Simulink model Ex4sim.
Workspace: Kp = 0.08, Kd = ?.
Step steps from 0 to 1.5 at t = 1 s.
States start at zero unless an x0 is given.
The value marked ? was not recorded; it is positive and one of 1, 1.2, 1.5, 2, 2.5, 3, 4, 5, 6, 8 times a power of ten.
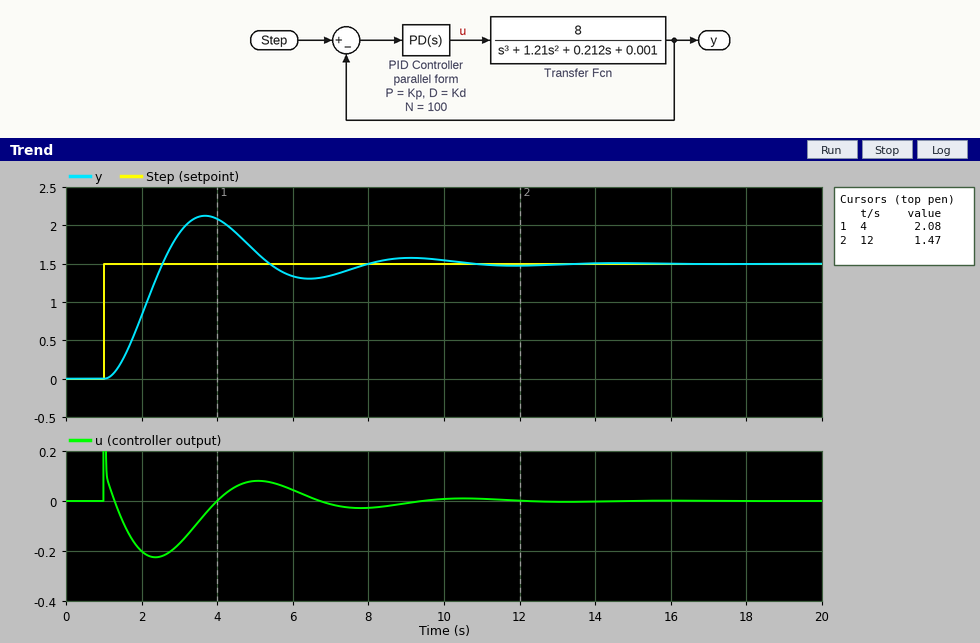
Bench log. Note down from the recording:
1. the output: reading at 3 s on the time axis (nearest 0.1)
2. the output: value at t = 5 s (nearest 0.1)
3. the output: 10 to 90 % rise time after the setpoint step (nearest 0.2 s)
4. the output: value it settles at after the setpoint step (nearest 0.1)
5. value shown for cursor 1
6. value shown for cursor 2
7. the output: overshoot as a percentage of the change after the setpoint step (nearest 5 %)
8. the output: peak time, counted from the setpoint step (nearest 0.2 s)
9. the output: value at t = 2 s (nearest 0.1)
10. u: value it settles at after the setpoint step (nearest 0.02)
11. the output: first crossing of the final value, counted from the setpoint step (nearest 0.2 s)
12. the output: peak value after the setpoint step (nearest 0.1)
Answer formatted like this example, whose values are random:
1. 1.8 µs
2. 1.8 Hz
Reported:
1. 1.9
2. 1.7
3. 1.0 s
4. 1.5
5. 2.08
6. 1.47
7. 40 %
8. 2.6 s
9. 0.8
10. 0.00
11. 1.6 s
12. 2.1
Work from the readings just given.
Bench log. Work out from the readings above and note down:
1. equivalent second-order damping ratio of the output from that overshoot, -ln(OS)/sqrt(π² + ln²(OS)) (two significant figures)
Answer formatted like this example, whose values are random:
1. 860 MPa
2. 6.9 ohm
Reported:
1. 0.28
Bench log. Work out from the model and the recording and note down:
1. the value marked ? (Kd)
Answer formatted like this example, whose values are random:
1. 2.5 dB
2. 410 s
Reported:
1. 0.2
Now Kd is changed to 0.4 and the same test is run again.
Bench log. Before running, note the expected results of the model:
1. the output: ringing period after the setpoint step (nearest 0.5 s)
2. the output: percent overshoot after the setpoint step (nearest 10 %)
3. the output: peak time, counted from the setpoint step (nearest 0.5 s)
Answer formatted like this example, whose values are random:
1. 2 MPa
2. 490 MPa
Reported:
1. 3.5 s
2. 40 %
3. 2.0 s
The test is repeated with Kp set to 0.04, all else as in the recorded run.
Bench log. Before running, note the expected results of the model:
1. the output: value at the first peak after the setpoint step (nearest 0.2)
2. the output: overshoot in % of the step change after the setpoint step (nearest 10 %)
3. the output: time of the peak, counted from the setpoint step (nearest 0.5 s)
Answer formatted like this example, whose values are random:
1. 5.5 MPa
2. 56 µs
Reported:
1. 1.8
2. 30 %
3. 2.5 s
